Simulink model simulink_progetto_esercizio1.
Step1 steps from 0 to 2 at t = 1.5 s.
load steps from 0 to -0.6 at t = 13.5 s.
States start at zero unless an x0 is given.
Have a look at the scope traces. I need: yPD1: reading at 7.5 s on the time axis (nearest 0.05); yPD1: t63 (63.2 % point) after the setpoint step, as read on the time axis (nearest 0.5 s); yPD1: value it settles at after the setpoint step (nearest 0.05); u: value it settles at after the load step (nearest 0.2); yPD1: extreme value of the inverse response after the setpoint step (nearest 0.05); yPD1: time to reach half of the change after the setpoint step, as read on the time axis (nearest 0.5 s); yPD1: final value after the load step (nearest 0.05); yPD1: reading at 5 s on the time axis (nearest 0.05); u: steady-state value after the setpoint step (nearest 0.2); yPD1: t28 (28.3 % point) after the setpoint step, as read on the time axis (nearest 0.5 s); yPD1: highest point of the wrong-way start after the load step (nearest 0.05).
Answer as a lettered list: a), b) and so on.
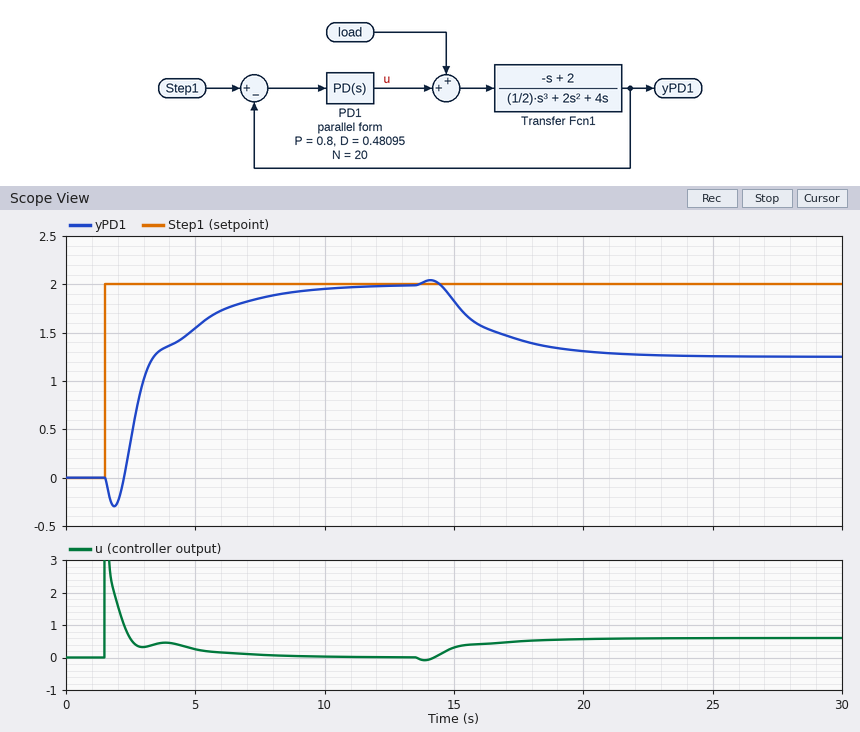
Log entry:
a) 1.85
b) 3.5 s
c) 2.00
d) 0.6
e) -0.30
f) 3.0 s
g) 1.25
h) 1.55
i) 0.0
j) 2.5 s
k) 2.05
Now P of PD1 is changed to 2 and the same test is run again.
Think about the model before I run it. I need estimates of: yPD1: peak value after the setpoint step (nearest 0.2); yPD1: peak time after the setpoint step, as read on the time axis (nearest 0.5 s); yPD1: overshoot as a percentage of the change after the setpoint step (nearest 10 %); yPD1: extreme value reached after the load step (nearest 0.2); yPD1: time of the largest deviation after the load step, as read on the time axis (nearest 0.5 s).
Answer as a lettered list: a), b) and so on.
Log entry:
a) 3.0
b) 3.5 s
c) 50 %
d) 1.6
e) 16.0 s
